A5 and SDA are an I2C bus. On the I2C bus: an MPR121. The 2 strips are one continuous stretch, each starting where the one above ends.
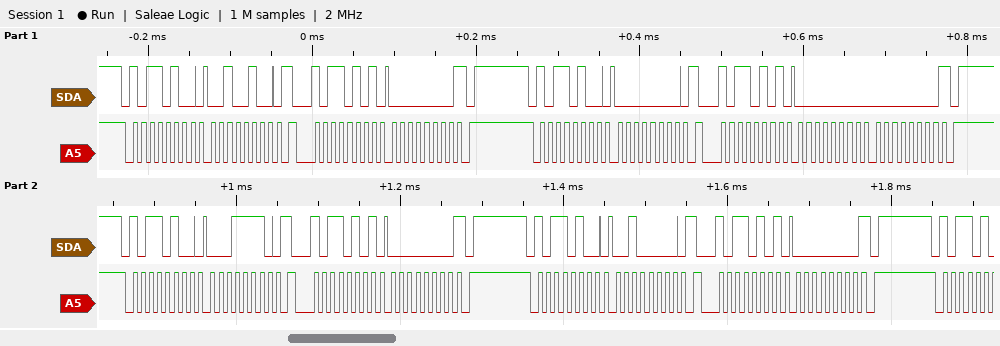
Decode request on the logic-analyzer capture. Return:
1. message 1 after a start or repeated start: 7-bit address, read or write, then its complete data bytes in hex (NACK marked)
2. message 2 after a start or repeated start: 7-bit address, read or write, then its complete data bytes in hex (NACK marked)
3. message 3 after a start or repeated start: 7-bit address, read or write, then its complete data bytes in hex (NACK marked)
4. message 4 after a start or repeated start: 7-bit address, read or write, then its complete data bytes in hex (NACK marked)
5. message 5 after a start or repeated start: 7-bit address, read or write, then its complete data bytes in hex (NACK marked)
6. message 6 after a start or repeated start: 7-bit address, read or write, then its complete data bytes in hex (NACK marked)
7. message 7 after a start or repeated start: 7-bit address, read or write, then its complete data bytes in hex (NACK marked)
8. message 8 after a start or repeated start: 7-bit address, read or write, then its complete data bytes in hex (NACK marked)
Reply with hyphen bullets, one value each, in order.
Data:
- 0x5A write: 24
- 0x5A read: 00 NACK
- 0x5A write: 00
- 0x5A read: 00 00 NACK
- 0x5A write: 1E
- 0x5A read: 00 NACK
- 0x5A write: 20
- 0x5A read: 00 NACK
